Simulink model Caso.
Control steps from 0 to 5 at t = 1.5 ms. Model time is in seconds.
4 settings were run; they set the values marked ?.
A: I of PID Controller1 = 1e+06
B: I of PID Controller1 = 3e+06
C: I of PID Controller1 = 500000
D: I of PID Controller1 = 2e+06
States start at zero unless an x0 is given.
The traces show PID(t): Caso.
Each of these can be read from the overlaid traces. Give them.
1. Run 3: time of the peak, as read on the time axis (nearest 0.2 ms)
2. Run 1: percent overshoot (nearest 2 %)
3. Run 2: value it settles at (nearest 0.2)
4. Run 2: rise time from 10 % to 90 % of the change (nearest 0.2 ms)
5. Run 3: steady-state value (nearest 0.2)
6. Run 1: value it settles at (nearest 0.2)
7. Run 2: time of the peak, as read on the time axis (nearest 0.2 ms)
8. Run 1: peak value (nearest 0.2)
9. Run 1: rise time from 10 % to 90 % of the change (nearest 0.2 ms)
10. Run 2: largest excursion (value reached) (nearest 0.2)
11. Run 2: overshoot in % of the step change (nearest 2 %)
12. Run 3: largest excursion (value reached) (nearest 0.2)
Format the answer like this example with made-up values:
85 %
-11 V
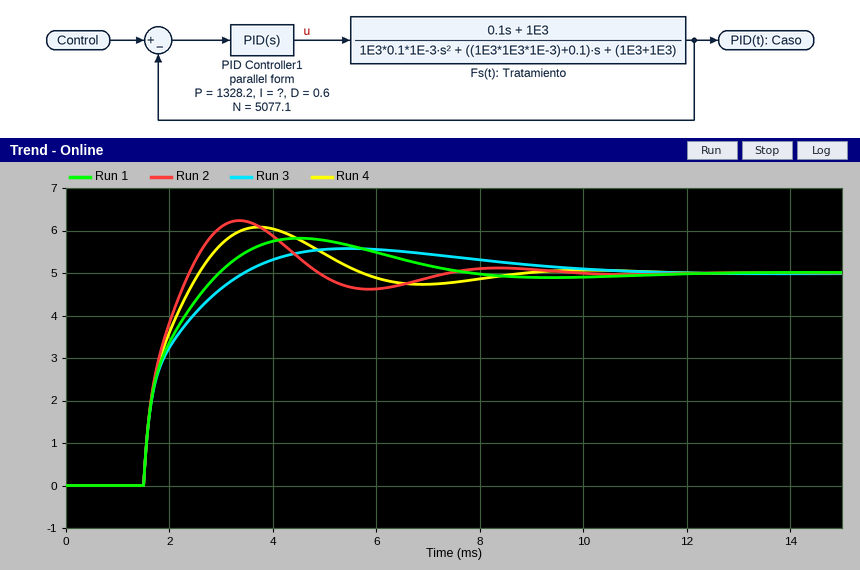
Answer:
5.4 ms
16 %
5.0
0.6 ms
5.0
5.0
3.4 ms
5.8
1.0 ms
6.2
24 %
5.6
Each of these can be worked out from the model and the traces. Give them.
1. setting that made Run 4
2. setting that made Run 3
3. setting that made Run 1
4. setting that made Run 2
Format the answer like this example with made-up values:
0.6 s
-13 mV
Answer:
D
C
A
B
